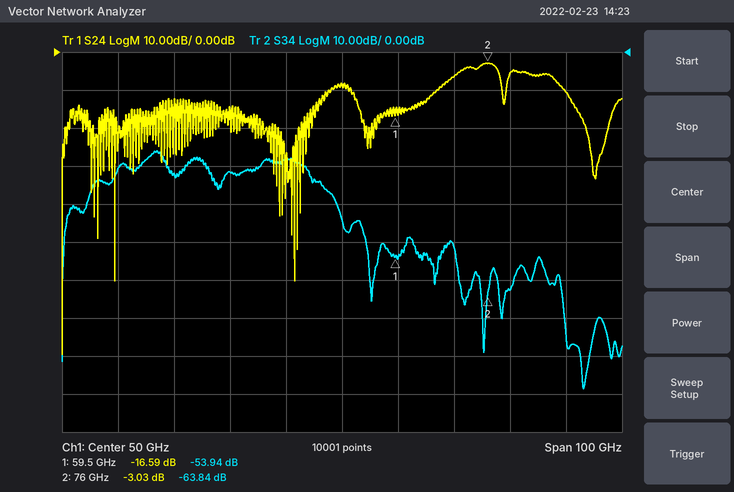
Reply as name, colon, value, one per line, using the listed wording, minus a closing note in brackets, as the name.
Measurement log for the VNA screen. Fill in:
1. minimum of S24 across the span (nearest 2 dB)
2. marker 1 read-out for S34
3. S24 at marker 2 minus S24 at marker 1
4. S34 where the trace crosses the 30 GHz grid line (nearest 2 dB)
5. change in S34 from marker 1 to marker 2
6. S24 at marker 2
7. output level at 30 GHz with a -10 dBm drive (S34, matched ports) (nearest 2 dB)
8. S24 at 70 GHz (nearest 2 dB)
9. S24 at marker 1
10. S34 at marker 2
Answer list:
minimum of S24 across the span: -80 dB
marker 1 read-out for S34: -53.94 dB
S24 at marker 2 minus S24 at marker 1: 13.56 dB
S34 where the trace crosses the 30 GHz grid line: -32 dB
change in S34 from marker 1 to marker 2: -9.90 dB
S24 at marker 2: -3.03 dB
output level at 30 GHz with a -10 dBm drive (S34, matched ports): -42 dBm
S24 at 70 GHz: -6 dB
S24 at marker 1: -16.59 dB
S34 at marker 2: -63.84 dB
